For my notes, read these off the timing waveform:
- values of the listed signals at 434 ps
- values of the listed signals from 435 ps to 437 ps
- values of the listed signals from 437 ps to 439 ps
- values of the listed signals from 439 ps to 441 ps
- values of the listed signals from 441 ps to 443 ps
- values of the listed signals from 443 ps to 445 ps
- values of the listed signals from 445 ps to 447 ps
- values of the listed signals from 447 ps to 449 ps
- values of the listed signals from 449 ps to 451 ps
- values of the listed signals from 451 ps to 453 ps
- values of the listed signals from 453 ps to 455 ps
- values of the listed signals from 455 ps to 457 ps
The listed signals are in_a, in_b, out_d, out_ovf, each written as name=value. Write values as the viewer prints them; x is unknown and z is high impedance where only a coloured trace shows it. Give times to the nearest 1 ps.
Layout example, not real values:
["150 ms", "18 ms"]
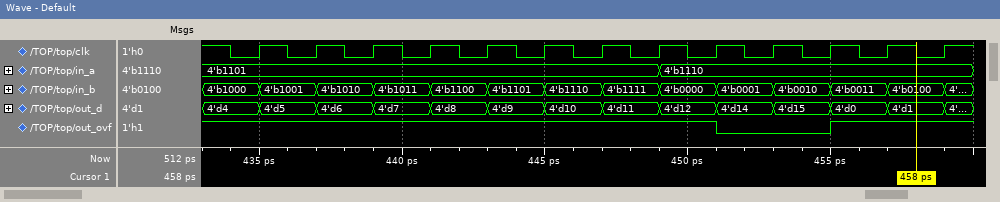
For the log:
["in_a=4'b1101, in_b=4'b1000, out_d=4'd4, out_ovf=1", "in_a=4'b1101, in_b=4'b1001, out_d=4'd5, out_ovf=1", "in_a=4'b1101, in_b=4'b1010, out_d=4'd6, out_ovf=1", "in_a=4'b1101, in_b=4'b1011, out_d=4'd7, out_ovf=1", "in_a=4'b1101, in_b=4'b1100, out_d=4'd8, out_ovf=1", "in_a=4'b1101, in_b=4'b1101, out_d=4'd9, out_ovf=1", "in_a=4'b1101, in_b=4'b1110, out_d=4'd10, out_ovf=1", "in_a=4'b1101, in_b=4'b1111, out_d=4'd11, out_ovf=1", "in_a=4'b1110, in_b=4'b0000, out_d=4'd12, out_ovf=1", "in_a=4'b1110, in_b=4'b0001, out_d=4'd14, out_ovf=0", "in_a=4'b1110, in_b=4'b0010, out_d=4'd15, out_ovf=0", "in_a=4'b1110, in_b=4'b0011, out_d=4'd0, out_ovf=1"]
